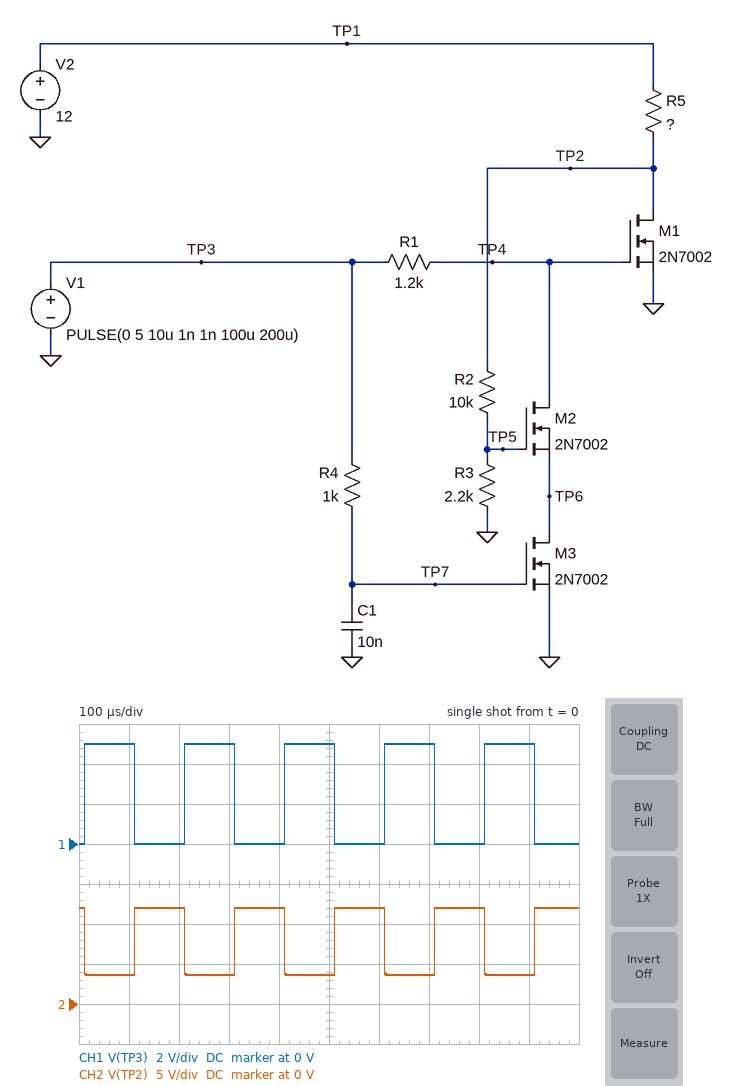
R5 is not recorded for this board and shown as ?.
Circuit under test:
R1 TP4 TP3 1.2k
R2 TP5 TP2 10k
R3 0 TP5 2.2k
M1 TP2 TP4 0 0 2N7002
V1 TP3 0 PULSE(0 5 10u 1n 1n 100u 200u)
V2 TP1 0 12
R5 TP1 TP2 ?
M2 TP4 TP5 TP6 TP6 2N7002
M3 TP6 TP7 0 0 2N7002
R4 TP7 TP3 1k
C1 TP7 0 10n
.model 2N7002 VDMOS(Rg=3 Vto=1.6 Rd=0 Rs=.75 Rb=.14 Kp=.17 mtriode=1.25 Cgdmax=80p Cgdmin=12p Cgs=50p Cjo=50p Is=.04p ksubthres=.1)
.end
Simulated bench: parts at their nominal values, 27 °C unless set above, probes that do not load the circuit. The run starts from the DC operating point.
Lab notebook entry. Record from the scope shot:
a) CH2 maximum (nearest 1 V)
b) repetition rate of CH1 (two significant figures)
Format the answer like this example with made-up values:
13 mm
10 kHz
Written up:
12 V
5.0 kHz
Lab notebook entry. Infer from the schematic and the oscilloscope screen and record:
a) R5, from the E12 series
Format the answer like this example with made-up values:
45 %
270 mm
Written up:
12 Ω
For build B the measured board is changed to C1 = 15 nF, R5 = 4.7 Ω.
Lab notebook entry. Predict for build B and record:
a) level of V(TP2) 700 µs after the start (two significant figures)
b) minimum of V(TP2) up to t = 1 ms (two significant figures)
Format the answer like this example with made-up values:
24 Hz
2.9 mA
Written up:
12 V
8.7 V
